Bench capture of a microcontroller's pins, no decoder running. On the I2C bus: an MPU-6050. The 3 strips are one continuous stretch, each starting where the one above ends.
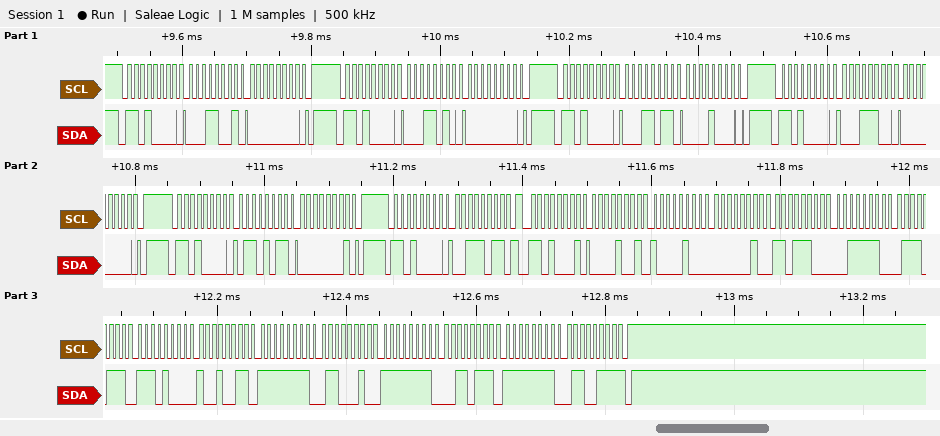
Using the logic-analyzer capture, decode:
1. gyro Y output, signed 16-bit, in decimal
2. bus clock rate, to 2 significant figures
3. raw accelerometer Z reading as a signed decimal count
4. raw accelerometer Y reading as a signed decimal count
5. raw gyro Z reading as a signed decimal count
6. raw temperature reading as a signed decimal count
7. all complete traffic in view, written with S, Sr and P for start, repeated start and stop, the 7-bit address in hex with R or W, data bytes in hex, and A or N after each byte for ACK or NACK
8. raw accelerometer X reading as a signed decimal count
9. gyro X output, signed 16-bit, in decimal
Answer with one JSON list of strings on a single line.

["-201", "100 kHz", "15991", "732", "-153", "-5997", "S 68W A 19 A 00 A P S 68W A 1A A 00 A P S 68W A 1B A 08 A P S 68W A 1C A 00 A P S 68W A 6B A 01 A P S 68W A 3B A Sr 68R A 09 A 84 A 02 A DC A 3E A 77 A E8 A 93 A FF A 62 A FF A 37 A FF A 67 N P", "2436", "-158"]
